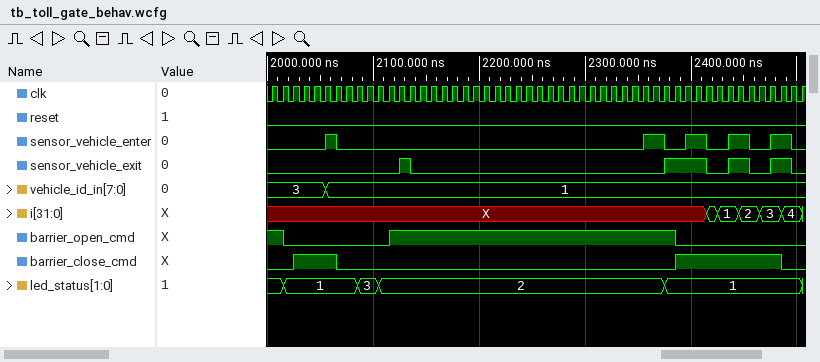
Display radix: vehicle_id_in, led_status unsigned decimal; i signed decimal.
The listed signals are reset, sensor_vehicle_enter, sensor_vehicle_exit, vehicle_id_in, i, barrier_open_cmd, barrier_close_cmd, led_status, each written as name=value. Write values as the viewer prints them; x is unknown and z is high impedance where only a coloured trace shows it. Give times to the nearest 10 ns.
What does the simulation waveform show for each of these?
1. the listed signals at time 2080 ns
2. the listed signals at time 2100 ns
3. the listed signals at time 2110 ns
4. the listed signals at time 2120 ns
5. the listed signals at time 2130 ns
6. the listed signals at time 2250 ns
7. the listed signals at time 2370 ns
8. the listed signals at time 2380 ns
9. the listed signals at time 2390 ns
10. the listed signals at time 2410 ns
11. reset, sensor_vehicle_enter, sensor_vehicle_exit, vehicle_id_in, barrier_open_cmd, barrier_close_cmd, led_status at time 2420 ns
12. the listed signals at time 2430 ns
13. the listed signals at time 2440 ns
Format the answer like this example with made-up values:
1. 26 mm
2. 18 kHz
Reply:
1. reset=0, sensor_vehicle_enter=0, sensor_vehicle_exit=0, vehicle_id_in=1, i=X, barrier_open_cmd=0, barrier_close_cmd=0, led_status=1
2. reset=0, sensor_vehicle_enter=0, sensor_vehicle_exit=0, vehicle_id_in=1, i=X, barrier_open_cmd=0, barrier_close_cmd=0, led_status=3
3. reset=0, sensor_vehicle_enter=0, sensor_vehicle_exit=0, vehicle_id_in=1, i=X, barrier_open_cmd=0, barrier_close_cmd=0, led_status=2
4. reset=0, sensor_vehicle_enter=0, sensor_vehicle_exit=0, vehicle_id_in=1, i=X, barrier_open_cmd=1, barrier_close_cmd=0, led_status=2
5. reset=0, sensor_vehicle_enter=0, sensor_vehicle_exit=1, vehicle_id_in=1, i=X, barrier_open_cmd=1, barrier_close_cmd=0, led_status=2
6. reset=0, sensor_vehicle_enter=0, sensor_vehicle_exit=0, vehicle_id_in=1, i=X, barrier_open_cmd=1, barrier_close_cmd=0, led_status=2
7. reset=0, sensor_vehicle_enter=1, sensor_vehicle_exit=0, vehicle_id_in=1, i=X, barrier_open_cmd=1, barrier_close_cmd=0, led_status=2
8. reset=0, sensor_vehicle_enter=0, sensor_vehicle_exit=1, vehicle_id_in=1, i=X, barrier_open_cmd=1, barrier_close_cmd=0, led_status=1
9. reset=0, sensor_vehicle_enter=0, sensor_vehicle_exit=1, vehicle_id_in=1, i=X, barrier_open_cmd=0, barrier_close_cmd=1, led_status=1
10. reset=0, sensor_vehicle_enter=1, sensor_vehicle_exit=1, vehicle_id_in=1, i=X, barrier_open_cmd=0, barrier_close_cmd=1, led_status=1
11. reset=0, sensor_vehicle_enter=0, sensor_vehicle_exit=0, vehicle_id_in=1, barrier_open_cmd=0, barrier_close_cmd=1, led_status=1
12. reset=0, sensor_vehicle_enter=0, sensor_vehicle_exit=0, vehicle_id_in=1, i=1, barrier_open_cmd=0, barrier_close_cmd=1, led_status=1
13. reset=0, sensor_vehicle_enter=1, sensor_vehicle_exit=1, vehicle_id_in=1, i=1, barrier_open_cmd=0, barrier_close_cmd=1, led_status=1
